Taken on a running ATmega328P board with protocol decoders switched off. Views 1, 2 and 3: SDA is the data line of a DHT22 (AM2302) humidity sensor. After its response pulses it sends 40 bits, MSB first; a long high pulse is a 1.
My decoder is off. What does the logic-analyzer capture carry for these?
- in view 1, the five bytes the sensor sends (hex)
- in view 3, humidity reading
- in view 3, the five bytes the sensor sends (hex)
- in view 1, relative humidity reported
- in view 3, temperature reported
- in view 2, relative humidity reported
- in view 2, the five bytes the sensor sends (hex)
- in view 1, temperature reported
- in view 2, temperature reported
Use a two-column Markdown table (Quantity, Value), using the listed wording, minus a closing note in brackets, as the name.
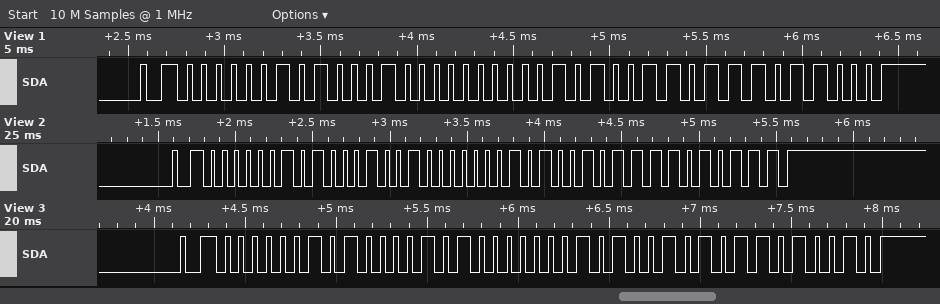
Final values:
| Quantity | Value |
|---|---|
| in view 1, the five bytes the sensor sends | 02 88 01 4D D8 |
| in view 3, humidity reading | 64.5 % |
| in view 3, the five bytes the sensor sends | 02 85 01 4A D2 |
| in view 1, relative humidity reported | 64.8 % |
| in view 3, temperature reported | 33.0 °C |
| in view 2, relative humidity reported | 64.9 % |
| in view 2, the five bytes the sensor sends | 02 89 01 4B D7 |
| in view 1, temperature reported | 33.3 °C |
| in view 2, temperature reported | 33.1 °C |
